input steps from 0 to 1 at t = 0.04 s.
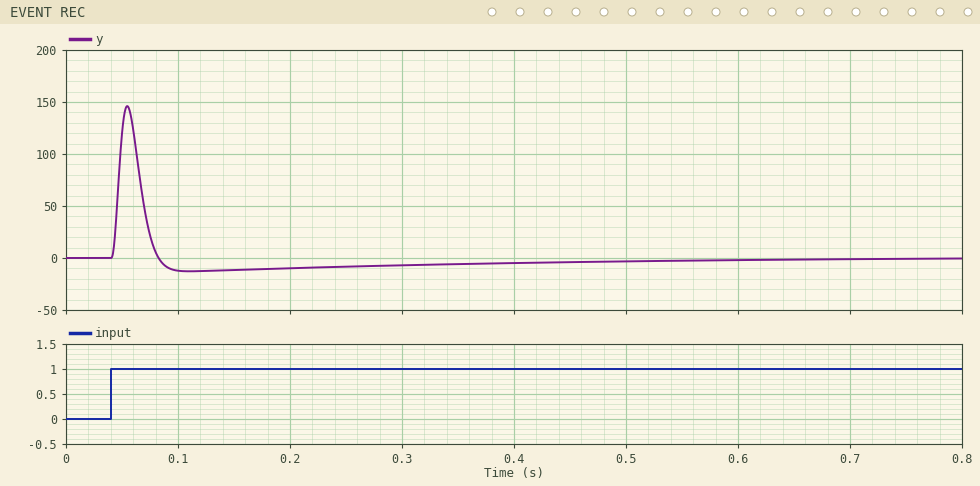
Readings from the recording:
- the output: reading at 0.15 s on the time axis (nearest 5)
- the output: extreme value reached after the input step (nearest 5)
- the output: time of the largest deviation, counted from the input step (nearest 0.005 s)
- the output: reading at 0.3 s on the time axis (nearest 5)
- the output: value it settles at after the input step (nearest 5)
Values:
-10
145
0.015 s
-5
0
